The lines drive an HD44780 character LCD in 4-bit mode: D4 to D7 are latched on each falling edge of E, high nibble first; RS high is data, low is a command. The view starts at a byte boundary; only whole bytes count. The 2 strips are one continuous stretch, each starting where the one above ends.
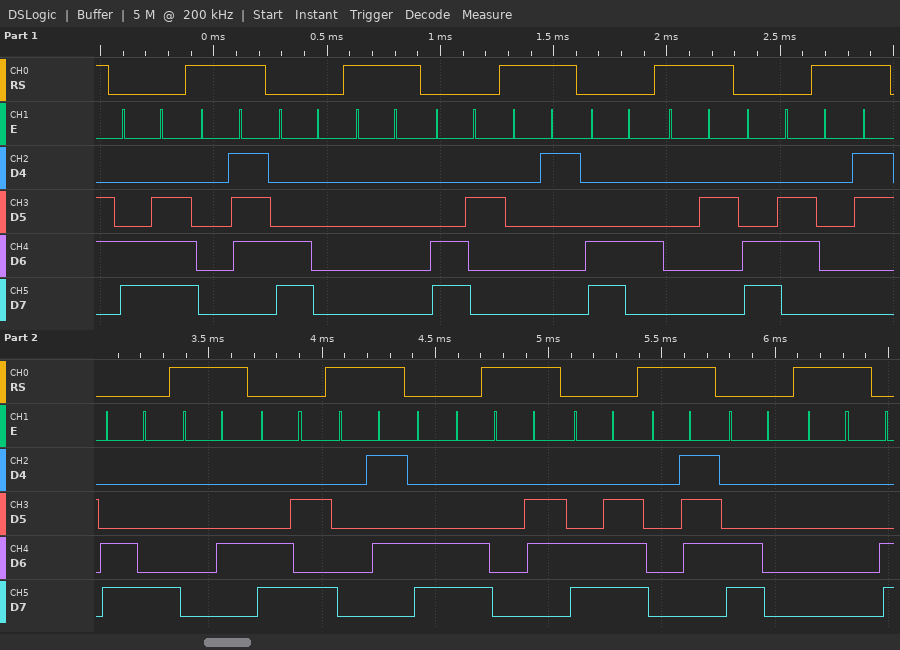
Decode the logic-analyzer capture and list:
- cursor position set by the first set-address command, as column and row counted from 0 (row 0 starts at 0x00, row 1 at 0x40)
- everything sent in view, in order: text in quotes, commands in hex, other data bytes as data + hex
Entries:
column 14, row 1
0xCE data 07 0xC0 data 00 0xC2 data 01 0xC4 data 02 0xC6 data 03 0xC8 data 04 0xCA data 05 0xCC data 06 0xCE data 07 0xC0 data 00
